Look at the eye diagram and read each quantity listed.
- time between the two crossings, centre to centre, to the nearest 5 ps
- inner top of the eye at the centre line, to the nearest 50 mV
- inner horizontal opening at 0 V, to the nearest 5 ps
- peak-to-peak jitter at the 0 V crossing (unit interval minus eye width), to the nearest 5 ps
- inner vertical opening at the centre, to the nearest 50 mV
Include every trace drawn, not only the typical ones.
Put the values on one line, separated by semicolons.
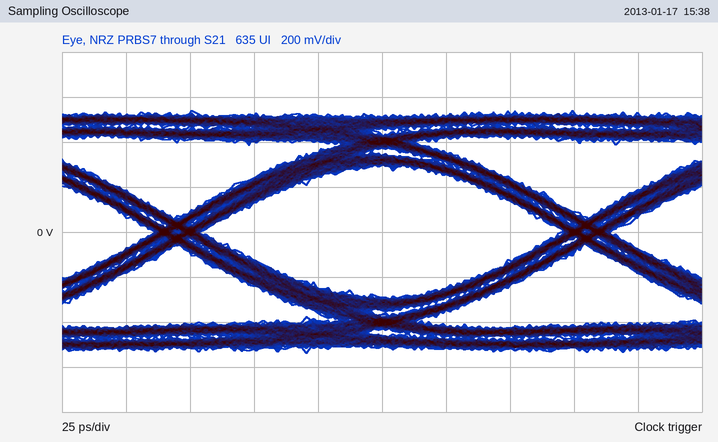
160 ps; 300 mV; 140 ps; 20 ps; 600 mV
